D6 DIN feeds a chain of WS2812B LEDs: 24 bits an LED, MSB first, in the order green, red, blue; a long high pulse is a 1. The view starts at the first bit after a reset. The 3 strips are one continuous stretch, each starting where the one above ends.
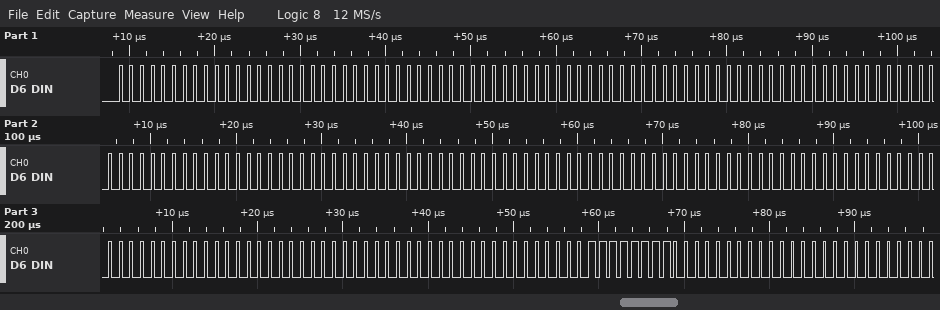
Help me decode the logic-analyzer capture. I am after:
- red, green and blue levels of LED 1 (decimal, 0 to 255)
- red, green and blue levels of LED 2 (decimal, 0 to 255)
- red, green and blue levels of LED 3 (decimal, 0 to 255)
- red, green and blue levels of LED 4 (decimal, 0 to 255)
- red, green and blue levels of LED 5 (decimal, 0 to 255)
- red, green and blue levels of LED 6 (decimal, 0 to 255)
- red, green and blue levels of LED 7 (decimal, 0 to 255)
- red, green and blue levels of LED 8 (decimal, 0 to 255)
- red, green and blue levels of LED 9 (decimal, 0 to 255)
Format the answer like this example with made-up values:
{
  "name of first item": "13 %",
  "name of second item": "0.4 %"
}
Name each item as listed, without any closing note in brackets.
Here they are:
{
  "red, green and blue levels of LED 1": "0, 0, 0",
  "red, green and blue levels of LED 2": "0, 0, 0",
  "red, green and blue levels of LED 3": "0, 0, 0",
  "red, green and blue levels of LED 4": "0, 0, 0",
  "red, green and blue levels of LED 5": "0, 0, 0",
  "red, green and blue levels of LED 6": "0, 0, 0",
  "red, green and blue levels of LED 7": "0, 0, 0",
  "red, green and blue levels of LED 8": "0, 0, 0",
  "red, green and blue levels of LED 9": "255, 0, 0"
}
